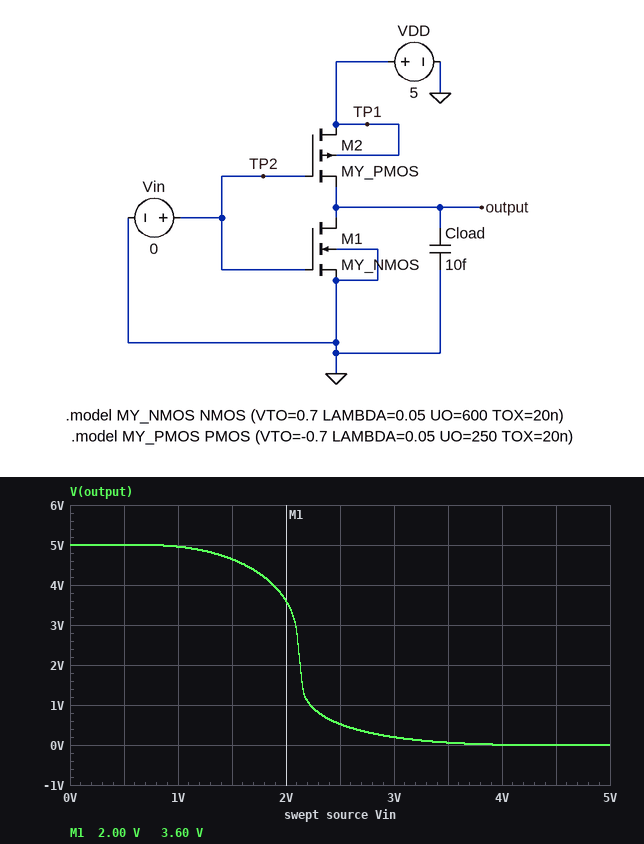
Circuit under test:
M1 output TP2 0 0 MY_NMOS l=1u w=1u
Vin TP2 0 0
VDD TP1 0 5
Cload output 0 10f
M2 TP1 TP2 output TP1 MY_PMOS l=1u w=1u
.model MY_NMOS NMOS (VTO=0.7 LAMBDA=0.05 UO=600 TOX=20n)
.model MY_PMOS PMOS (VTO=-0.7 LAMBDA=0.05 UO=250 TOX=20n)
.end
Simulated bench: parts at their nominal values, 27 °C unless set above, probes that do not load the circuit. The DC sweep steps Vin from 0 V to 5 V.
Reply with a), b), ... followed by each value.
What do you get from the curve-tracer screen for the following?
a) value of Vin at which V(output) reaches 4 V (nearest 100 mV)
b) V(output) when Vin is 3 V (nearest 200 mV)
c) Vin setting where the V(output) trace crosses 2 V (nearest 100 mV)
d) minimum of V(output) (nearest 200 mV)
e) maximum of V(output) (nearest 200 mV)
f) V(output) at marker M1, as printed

a) 1.9 V
b) 200 mV
c) 2.1 V
d) 0 V
e) 5.0 V
f) 3.60 V
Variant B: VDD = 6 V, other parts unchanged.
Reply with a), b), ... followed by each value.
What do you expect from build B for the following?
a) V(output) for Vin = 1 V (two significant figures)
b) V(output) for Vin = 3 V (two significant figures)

a) 6.0 V
b) 690 mV
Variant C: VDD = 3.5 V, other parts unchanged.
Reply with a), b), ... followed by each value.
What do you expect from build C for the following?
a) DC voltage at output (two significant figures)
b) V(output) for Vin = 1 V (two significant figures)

a) 3.5 V
b) 3.4 V
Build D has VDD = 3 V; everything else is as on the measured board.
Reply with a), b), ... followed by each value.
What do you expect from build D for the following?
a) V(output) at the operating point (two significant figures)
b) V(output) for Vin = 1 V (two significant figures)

a) 3.0 V
b) 2.9 V
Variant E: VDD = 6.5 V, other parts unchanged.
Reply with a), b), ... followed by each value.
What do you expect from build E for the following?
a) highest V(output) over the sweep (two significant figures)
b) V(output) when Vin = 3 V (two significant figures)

a) 6.5 V
b) 1.1 V
